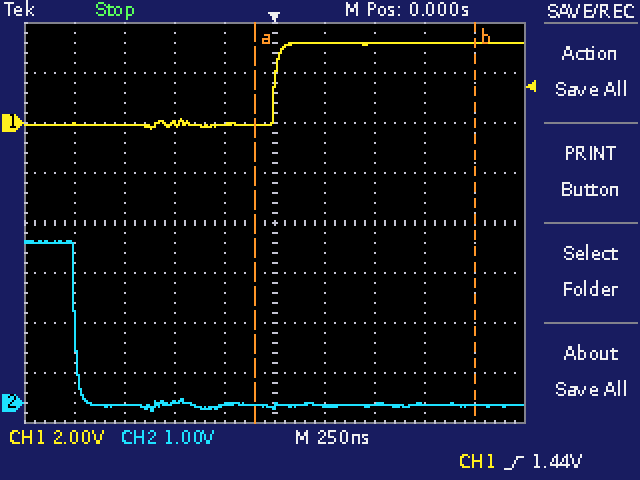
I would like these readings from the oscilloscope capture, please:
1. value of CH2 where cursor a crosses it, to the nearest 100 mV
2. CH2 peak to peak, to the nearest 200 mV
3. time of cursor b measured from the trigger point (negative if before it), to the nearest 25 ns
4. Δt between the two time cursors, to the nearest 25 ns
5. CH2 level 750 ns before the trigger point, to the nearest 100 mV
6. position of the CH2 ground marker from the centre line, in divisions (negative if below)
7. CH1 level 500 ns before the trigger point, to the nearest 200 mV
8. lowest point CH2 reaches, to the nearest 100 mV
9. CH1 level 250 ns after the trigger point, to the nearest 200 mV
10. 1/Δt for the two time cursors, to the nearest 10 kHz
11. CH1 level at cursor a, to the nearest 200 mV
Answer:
0.0 V
3.4 V
+1.000 µs
1.100 µs
0.0 V
-3.6 div
0.0 V
-200 mV
3.2 V
910 kHz
0.0 V
